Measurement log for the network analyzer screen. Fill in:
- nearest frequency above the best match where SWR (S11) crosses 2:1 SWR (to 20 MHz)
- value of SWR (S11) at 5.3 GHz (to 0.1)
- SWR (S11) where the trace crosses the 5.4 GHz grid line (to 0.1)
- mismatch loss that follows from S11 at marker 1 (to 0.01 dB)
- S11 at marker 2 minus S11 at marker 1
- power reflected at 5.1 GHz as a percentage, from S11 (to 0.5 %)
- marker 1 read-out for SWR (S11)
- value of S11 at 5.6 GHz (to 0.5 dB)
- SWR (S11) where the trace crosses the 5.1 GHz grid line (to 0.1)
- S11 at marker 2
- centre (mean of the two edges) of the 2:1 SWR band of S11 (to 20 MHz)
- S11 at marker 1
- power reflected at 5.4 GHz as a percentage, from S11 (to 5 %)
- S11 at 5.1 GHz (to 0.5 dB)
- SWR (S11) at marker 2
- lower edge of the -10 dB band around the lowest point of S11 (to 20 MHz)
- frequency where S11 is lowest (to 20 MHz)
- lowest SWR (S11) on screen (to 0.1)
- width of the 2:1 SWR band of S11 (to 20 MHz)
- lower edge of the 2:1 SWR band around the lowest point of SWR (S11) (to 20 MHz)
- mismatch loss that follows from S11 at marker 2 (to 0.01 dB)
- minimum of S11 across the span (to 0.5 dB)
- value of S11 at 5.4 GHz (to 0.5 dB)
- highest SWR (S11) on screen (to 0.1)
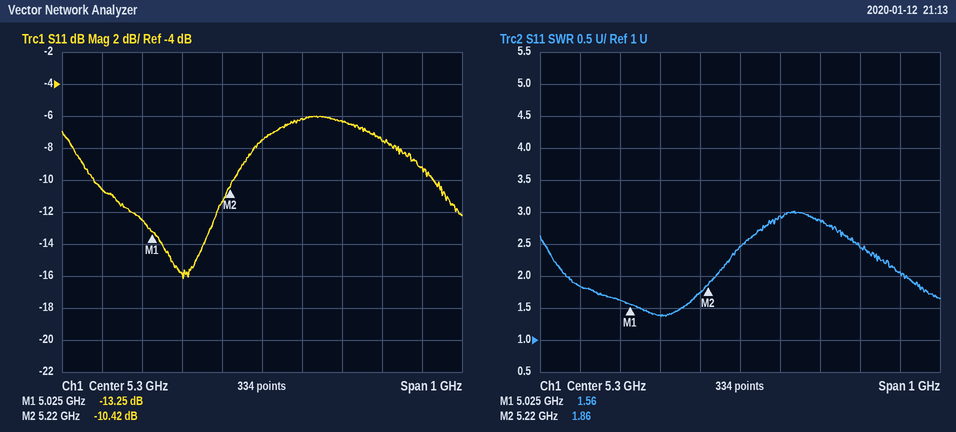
5.24 GHz
2.5
2.9
0.21 dB
2.83 dB
2.5 %
1.56
-7.5 dB
1.4
-10.42 dB
5.06 GHz
-13.25 dB
25 %
-16.0 dB
1.86
4.88 GHz
5.10 GHz
1.4
380 MHz
4.86 GHz
0.41 dB
-16.0 dB
-6.0 dB
3.0
